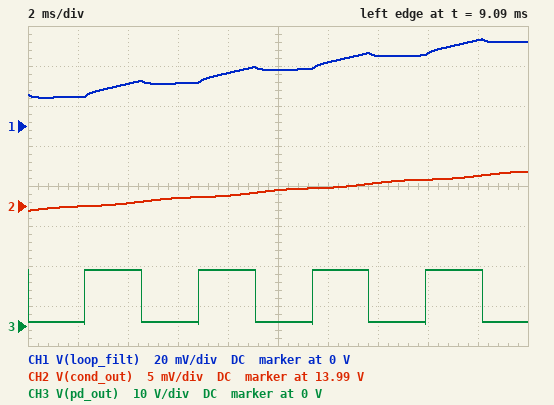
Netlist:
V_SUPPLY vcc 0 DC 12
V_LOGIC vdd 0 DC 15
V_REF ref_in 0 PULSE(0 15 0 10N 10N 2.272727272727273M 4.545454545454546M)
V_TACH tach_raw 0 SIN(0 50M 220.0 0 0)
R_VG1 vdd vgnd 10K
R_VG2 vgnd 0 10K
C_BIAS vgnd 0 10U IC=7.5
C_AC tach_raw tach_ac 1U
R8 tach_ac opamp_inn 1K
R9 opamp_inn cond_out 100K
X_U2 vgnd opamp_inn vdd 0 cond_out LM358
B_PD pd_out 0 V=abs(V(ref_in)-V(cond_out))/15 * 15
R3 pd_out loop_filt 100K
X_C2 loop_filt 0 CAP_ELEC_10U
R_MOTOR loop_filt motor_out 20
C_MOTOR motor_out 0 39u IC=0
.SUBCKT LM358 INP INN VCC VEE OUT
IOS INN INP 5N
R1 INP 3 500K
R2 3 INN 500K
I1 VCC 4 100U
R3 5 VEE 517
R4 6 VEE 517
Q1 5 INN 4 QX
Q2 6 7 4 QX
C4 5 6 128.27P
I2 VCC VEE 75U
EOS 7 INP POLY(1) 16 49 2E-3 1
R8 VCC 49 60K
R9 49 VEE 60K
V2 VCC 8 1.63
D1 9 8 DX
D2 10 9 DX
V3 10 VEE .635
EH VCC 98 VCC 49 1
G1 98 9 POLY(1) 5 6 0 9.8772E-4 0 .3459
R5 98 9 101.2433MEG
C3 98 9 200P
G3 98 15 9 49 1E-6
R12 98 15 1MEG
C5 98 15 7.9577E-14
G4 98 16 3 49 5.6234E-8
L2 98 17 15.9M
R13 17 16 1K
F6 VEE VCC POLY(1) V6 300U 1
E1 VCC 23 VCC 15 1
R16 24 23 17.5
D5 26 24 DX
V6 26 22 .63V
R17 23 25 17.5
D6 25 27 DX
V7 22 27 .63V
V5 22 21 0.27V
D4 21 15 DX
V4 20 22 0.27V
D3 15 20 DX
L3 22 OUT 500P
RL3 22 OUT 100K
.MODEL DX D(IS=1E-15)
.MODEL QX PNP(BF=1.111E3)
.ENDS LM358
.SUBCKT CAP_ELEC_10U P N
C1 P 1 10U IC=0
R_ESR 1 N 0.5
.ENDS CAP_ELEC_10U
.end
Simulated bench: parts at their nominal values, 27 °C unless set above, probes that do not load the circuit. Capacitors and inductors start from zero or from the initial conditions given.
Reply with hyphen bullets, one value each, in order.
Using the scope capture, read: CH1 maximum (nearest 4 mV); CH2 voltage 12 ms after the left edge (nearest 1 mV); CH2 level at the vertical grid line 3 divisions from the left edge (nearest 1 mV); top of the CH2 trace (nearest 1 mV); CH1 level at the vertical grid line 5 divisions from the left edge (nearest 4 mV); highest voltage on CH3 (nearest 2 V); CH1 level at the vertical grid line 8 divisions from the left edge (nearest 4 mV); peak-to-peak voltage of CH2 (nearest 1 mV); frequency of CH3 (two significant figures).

- 44 mV
- 13.992 V
- 13.991 V
- 13.994 V
- 28 mV
- 14 V
- 36 mV
- 5 mV
- 220 Hz
